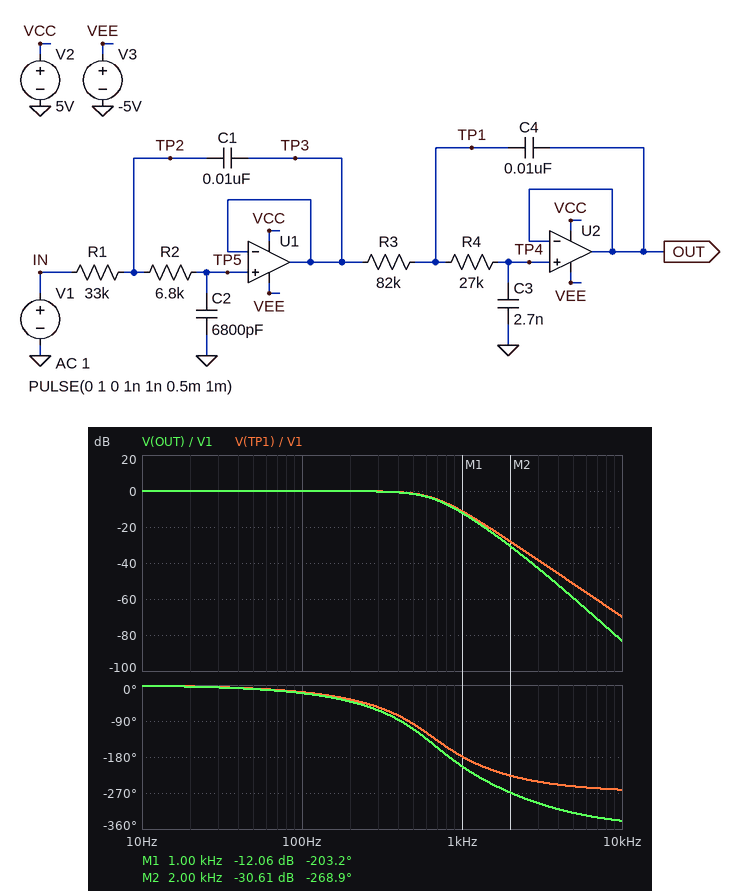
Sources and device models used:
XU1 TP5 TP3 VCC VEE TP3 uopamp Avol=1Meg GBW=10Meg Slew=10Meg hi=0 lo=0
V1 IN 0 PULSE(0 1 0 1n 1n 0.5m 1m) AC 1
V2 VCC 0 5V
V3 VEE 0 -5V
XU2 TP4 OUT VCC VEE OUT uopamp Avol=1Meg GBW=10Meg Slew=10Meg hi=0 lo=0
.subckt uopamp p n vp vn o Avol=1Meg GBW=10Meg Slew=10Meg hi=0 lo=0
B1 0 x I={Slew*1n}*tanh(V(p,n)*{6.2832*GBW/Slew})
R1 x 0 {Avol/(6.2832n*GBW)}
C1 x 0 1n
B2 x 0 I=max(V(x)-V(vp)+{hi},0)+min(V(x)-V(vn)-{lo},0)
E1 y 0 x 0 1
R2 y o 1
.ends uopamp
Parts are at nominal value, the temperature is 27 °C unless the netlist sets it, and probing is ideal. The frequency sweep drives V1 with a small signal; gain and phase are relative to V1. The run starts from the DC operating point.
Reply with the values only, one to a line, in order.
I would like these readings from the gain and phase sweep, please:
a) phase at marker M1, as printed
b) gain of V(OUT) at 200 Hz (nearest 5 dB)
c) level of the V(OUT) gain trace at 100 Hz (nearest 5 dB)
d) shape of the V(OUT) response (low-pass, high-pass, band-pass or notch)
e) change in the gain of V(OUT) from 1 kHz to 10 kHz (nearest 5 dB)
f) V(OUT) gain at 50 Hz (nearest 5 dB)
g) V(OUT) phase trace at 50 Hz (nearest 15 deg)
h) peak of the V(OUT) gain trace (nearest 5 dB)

-203.2 deg
0 dB
0 dB
low-pass
-70 dB
0 dB
-15 deg
0 dB
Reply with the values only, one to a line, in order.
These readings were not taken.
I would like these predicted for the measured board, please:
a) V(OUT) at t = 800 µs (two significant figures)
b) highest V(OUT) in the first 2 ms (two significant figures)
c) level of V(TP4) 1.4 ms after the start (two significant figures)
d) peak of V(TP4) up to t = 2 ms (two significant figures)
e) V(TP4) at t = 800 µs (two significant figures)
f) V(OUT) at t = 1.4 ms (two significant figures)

690 mV
700 mV
370 mV
700 mV
690 mV
370 mV
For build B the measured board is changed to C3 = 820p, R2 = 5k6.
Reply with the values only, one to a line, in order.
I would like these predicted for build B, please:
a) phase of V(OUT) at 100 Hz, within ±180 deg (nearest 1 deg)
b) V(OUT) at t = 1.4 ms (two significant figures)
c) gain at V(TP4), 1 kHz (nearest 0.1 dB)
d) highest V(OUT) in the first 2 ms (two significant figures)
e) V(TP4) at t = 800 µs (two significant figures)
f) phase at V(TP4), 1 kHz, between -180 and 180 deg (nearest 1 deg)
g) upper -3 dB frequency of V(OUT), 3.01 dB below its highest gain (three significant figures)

-13 deg
580 mV
-0.7 dB
1.1 V
750 mV
-136 deg
1.23 kHz
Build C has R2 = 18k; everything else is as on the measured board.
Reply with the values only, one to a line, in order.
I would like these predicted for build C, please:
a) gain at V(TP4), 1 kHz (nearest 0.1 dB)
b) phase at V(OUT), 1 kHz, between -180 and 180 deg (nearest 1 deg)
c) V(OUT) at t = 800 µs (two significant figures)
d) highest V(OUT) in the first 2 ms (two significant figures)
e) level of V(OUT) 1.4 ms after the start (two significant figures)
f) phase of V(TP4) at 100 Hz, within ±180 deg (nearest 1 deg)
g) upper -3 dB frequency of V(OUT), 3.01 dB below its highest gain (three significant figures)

-14.3 dB
128 deg
620 mV
660 mV
400 mV
-23 deg
562 Hz
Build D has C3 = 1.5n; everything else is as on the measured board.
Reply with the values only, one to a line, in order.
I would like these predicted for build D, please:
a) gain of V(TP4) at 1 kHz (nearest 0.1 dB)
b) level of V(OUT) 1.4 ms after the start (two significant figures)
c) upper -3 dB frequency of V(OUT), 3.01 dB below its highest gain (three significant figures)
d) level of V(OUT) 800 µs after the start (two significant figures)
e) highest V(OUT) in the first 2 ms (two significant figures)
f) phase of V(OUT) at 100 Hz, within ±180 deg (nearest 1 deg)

-5.5 dB
280 mV
872 Hz
860 mV
890 mV
-16 deg
